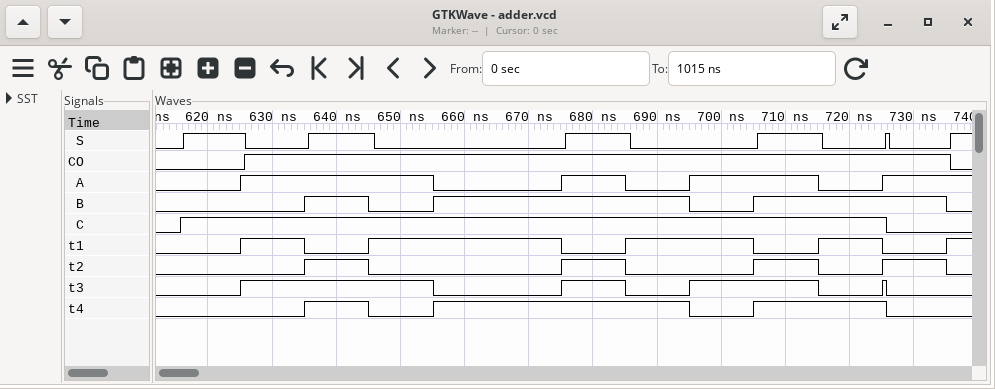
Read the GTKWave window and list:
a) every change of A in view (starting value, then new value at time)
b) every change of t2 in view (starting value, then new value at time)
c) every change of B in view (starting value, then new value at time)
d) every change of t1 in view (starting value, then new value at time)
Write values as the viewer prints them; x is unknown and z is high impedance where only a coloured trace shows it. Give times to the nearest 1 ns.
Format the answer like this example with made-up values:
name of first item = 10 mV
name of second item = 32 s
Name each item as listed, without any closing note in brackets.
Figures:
every change of A in view = 0, 1 at 625 ns, 0 at 655 ns, 1 at 675 ns, 0 at 685 ns, 1 at 695 ns, 0 at 715 ns, 1 at 725 ns
every change of t2 in view = 0, 1 at 635 ns, 0 at 645 ns, 1 at 675 ns, 0 at 685 ns, 1 at 705 ns, 0 at 715 ns, 1 at 725 ns, 0 at 735 ns
every change of B in view = 0, 1 at 635 ns, 0 at 645 ns, 1 at 655 ns, 0 at 695 ns, 1 at 705 ns, 0 at 735 ns
every change of t1 in view = 0, 1 at 625 ns, 0 at 635 ns, 1 at 645 ns, 0 at 675 ns, 1 at 685 ns, 0 at 705 ns, 1 at 715 ns, 0 at 725 ns, 1 at 735 ns
